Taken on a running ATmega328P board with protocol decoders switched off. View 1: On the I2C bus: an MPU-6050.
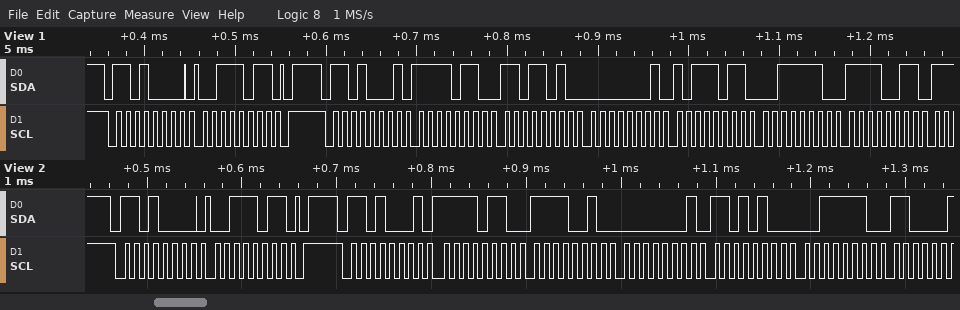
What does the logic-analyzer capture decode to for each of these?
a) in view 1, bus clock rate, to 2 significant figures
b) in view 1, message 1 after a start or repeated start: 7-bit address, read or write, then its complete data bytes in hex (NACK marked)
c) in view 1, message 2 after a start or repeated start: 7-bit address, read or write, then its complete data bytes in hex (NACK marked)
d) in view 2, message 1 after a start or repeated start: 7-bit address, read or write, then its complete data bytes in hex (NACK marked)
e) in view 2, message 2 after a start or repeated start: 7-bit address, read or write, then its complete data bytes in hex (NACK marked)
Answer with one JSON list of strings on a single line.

["100 kHz", "0x68 write: 3B", "0x68 read: F6 DA 01 BB 3E F3", "0x68 write: 3B", "0x68 read: F6 F2 01 D4 3E"]
